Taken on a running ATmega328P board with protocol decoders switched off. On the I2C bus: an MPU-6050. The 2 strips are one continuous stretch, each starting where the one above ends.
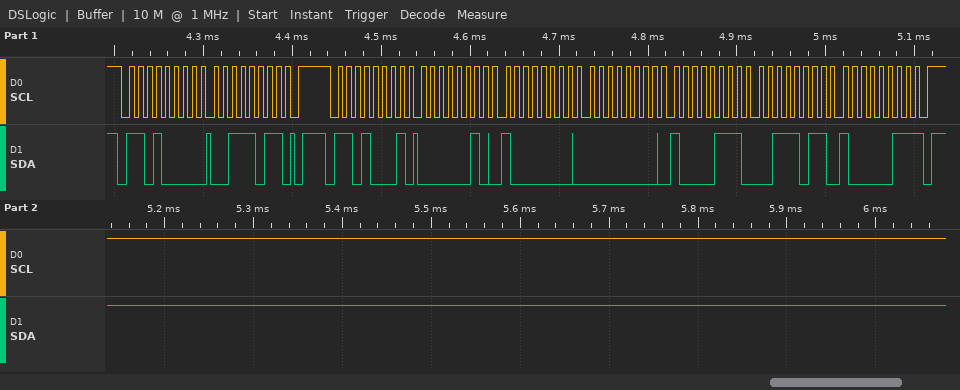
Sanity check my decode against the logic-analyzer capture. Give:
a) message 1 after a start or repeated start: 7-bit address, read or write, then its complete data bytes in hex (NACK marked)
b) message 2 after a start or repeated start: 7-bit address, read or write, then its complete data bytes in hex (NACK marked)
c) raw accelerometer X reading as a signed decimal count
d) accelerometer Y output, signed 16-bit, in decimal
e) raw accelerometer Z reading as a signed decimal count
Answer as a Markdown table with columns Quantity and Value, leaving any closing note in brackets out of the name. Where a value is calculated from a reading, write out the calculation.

| Quantity | Value |
|---|---|
| message 1 after a start or repeated start: 7-bit address, read or write, then its complete data bytes in hex | 0x68 write: 3B |
| message 2 after a start or repeated start: 7-bit address, read or write, then its complete data bytes in hex | 0x68 read: 02 80 00 87 3B 83 NACK |
| raw accelerometer X reading as a signed decimal count | 0x0280 = 640 |
| accelerometer Y output, signed 16-bit, in decimal | 0x0087 = 135 |
| raw accelerometer Z reading as a signed decimal count | 0x3B83 = 15235 |
